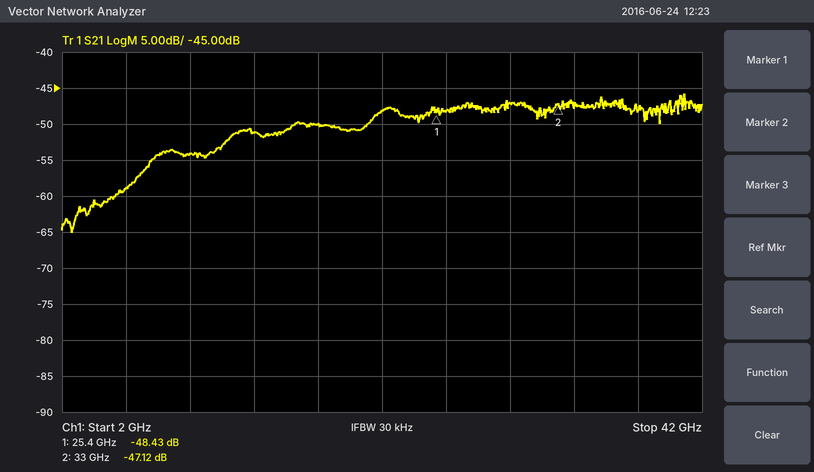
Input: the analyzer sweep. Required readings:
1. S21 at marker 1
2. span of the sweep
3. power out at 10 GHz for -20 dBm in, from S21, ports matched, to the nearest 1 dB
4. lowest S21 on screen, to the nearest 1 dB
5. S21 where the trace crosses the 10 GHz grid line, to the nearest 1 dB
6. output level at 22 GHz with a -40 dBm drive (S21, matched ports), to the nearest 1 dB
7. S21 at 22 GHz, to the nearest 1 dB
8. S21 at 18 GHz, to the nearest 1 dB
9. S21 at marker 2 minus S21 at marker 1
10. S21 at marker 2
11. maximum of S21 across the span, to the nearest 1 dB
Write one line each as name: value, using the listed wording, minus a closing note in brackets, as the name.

S21 at marker 1: -48.43 dB
span of the sweep: 40 GHz
power out at 10 GHz for -20 dBm in, from S21, ports matched, to the nearest 1 dB: -74 dBm
lowest S21 on screen, to the nearest 1 dB: -65 dB
S21 where the trace crosses the 10 GHz grid line, to the nearest 1 dB: -54 dB
output level at 22 GHz with a -40 dBm drive (S21, matched ports), to the nearest 1 dB: -88 dBm
S21 at 22 GHz, to the nearest 1 dB: -48 dB
S21 at 18 GHz, to the nearest 1 dB: -50 dB
S21 at marker 2 minus S21 at marker 1: 1.31 dB
S21 at marker 2: -47.12 dB
maximum of S21 across the span, to the nearest 1 dB: -46 dB
